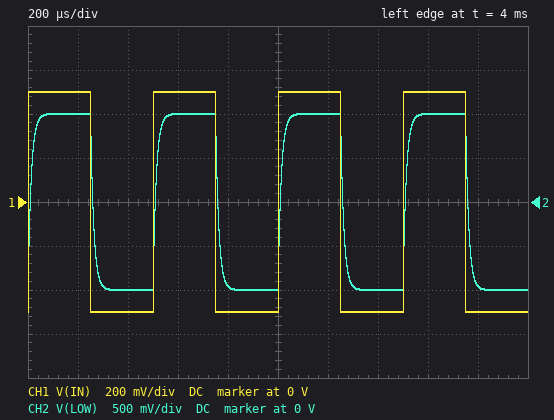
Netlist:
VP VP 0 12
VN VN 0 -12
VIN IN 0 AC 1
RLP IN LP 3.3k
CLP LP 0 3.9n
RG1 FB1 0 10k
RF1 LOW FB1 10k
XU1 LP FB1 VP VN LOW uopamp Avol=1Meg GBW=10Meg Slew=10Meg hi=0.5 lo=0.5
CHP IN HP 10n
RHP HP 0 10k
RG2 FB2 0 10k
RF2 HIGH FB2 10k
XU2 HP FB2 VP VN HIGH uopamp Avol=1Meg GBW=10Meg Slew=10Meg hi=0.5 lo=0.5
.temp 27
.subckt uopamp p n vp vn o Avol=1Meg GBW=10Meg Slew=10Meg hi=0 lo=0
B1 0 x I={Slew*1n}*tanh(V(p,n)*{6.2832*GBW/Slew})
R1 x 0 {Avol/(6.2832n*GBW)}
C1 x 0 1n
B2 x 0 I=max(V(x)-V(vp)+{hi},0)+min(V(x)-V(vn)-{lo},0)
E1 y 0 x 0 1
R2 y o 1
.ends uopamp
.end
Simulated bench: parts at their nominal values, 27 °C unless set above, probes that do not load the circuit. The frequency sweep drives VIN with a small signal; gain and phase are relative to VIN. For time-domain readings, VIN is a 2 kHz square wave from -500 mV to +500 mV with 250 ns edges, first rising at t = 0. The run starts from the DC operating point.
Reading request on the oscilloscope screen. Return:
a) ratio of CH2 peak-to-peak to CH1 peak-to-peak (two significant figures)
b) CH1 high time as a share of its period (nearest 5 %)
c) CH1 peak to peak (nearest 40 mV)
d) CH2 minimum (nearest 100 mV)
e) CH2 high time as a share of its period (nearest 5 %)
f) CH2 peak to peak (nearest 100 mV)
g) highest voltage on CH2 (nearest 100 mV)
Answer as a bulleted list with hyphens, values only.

- 2.0
- 50 %
- 1.00 V
- -1.0 V
- 50 %
- 2.0 V
- 1.0 V
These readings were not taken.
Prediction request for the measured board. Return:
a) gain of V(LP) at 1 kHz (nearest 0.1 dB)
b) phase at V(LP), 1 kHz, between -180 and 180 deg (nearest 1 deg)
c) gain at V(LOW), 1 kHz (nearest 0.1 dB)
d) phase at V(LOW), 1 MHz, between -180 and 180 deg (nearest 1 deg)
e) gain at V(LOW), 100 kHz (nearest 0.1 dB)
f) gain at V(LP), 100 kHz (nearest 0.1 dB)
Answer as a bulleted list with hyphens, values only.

- 0 dB
- -5 deg
- 6.0 dB
- -101 deg
- -12.2 dB
- -18.2 dB
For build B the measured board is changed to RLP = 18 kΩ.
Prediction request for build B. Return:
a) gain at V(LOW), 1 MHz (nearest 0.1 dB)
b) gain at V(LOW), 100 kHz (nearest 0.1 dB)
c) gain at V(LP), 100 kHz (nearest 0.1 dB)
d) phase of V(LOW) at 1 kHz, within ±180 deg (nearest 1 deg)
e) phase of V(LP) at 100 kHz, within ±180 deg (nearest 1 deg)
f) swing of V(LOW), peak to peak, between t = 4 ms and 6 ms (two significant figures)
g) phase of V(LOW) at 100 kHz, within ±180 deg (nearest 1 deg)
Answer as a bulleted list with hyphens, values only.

- -47.0 dB
- -26.9 dB
- -32.9 dB
- -24 deg
- -89 deg
- 1.9 V
- -90 deg
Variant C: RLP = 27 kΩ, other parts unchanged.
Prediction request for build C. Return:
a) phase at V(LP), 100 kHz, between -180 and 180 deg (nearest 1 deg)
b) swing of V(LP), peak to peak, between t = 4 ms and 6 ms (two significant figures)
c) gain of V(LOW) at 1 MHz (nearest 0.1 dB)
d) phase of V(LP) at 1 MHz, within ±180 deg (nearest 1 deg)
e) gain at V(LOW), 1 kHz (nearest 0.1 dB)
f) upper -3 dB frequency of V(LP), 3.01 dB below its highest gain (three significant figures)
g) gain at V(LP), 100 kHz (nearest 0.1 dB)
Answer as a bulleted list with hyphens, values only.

- -89 deg
- 830 mV
- -50.6 dB
- -90 deg
- 4.4 dB
- 1.51 kHz
- -36.4 dB
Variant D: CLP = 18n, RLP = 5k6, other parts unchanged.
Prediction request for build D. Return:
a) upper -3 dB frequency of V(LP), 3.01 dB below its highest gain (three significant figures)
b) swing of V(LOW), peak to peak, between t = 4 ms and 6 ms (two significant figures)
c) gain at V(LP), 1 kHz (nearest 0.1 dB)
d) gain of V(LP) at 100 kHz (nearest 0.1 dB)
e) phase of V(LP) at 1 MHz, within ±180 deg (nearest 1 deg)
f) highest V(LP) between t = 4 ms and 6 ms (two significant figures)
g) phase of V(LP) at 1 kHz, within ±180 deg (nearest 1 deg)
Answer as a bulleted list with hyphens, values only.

- 1.58 kHz
- 1.7 V
- -1.5 dB
- -36.0 dB
- -90 deg
- 420 mV
- -32 deg
